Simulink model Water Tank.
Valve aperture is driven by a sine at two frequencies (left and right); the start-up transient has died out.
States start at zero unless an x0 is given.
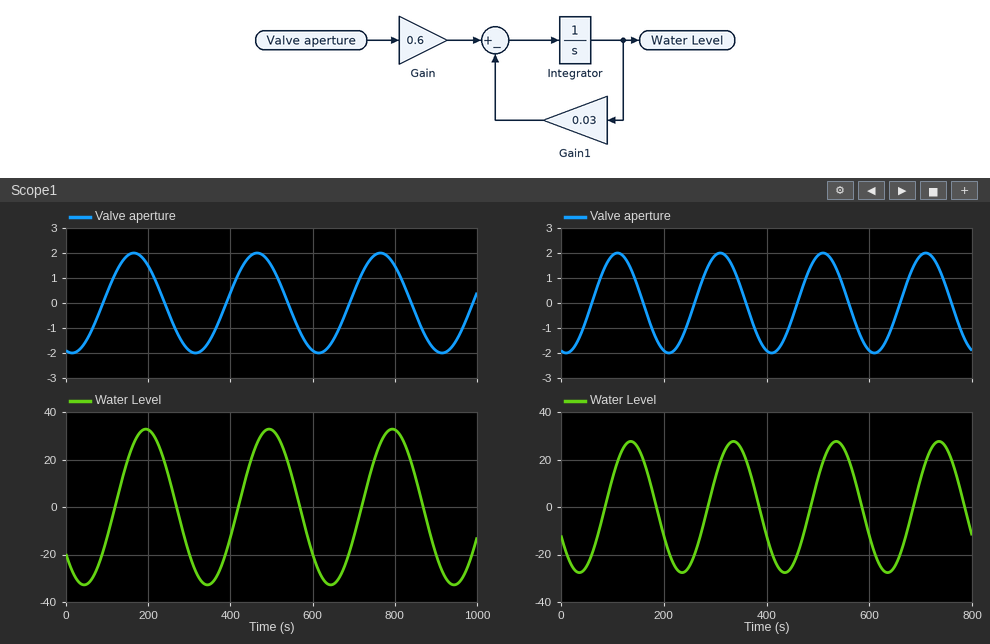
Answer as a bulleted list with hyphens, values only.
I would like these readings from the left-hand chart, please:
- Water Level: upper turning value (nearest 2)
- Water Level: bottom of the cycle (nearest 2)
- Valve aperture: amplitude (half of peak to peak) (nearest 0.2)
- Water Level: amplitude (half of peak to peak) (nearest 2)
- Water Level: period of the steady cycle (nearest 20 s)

- 32
- -32
- 2.0
- 32
- 300 s
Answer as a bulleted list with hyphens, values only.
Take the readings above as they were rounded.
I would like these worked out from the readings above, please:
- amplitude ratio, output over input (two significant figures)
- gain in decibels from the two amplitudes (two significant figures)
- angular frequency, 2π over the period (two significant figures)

- 16
- 24 dB
- 0.021 rad/s
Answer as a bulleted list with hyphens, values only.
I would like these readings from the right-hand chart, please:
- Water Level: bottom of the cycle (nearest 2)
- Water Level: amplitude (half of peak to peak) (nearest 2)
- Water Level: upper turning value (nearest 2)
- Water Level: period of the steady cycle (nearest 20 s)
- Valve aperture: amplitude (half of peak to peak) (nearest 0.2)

- -28
- 28
- 28
- 200 s
- 2.0
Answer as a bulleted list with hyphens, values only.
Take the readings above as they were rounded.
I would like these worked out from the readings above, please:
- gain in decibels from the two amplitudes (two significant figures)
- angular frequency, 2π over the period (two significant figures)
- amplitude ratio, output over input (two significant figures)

- 23 dB
- 0.031 rad/s
- 14
